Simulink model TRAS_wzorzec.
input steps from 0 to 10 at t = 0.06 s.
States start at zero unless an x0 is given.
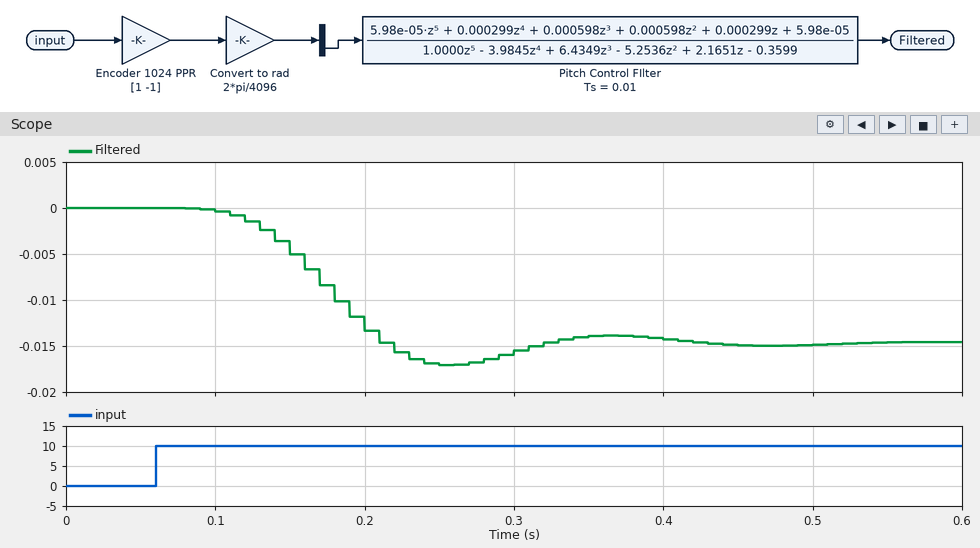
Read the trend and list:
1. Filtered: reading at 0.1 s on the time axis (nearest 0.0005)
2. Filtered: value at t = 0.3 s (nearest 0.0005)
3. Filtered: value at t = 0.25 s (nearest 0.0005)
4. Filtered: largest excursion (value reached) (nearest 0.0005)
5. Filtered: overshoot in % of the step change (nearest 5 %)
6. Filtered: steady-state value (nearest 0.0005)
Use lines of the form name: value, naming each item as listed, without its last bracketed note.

Filtered: reading at 0.1 s on the time axis: -0.0005
Filtered: value at t = 0.3 s: -0.0155
Filtered: value at t = 0.25 s: -0.0170
Filtered: largest excursion (value reached): -0.0170
Filtered: overshoot in % of the step change: 15 %
Filtered: steady-state value: -0.0145
